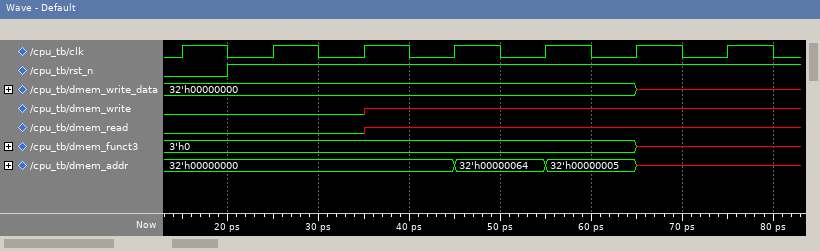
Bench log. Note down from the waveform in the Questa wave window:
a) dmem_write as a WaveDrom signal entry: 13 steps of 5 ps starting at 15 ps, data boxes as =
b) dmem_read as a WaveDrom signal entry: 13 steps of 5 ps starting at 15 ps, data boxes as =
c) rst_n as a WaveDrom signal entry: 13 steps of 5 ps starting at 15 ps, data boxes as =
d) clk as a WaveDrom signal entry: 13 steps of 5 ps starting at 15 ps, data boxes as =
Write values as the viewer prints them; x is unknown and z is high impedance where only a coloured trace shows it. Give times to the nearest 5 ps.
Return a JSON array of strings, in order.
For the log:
["{name: 'dmem_write', wave: '0...x........'}", "{name: 'dmem_read', wave: '0...x........'}", "{name: 'rst_n', wave: '01...........'}", "{name: 'clk', wave: '1010101010101'}"]
